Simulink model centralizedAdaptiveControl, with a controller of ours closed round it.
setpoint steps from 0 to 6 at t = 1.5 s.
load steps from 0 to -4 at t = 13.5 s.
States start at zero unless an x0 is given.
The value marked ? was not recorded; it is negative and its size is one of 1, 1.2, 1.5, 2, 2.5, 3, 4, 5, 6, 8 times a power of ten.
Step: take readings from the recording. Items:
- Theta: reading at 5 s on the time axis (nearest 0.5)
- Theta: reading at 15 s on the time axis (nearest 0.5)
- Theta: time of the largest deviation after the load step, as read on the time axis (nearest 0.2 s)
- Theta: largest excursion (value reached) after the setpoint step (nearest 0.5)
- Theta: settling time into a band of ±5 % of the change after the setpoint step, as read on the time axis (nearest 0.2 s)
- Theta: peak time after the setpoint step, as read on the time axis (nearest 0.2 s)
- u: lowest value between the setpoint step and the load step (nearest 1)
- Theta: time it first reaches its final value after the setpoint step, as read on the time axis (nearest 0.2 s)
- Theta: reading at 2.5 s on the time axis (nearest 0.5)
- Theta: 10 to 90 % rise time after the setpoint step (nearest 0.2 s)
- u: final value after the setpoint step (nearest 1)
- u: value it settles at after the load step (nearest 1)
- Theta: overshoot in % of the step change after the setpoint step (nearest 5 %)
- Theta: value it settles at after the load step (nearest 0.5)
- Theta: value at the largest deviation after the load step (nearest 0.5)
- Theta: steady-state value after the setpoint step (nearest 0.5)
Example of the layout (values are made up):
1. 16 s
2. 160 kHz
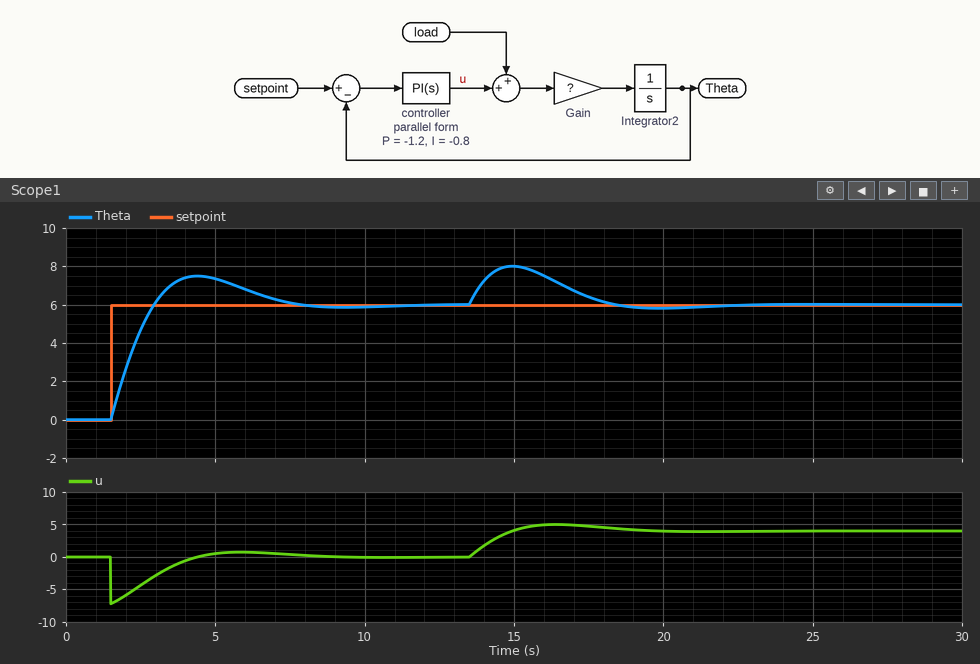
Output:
1. 7.5
2. 8.0
3. 15.0 s
4. 7.5
5. 7.0 s
6. 4.4 s
7. -7
8. 3.0 s
9. 4.5
10. 1.2 s
11. 0
12. 4
13. 25 %
14. 6.0
15. 8.0
16. 6.0
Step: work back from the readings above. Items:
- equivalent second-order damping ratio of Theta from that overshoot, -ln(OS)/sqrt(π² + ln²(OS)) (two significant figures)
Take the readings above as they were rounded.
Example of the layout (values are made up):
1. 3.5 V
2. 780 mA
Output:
1. 0.40
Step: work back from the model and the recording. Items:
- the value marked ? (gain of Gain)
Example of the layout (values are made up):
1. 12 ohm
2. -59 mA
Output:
1. -0.8
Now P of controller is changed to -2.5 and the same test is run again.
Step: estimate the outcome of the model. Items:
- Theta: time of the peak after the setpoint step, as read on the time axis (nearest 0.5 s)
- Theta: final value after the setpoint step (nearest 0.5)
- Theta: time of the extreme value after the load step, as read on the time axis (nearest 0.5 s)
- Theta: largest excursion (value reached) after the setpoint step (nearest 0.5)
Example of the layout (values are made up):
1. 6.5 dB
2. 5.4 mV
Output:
1. 4.0 s
2. 6.0
3. 14.5 s
4. 6.5
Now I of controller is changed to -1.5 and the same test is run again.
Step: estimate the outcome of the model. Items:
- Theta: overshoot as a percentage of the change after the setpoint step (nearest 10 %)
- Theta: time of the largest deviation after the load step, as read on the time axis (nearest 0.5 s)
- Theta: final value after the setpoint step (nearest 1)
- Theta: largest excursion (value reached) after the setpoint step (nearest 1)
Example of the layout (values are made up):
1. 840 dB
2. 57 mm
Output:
1. 30 %
2. 14.5 s
3. 6
4. 8
